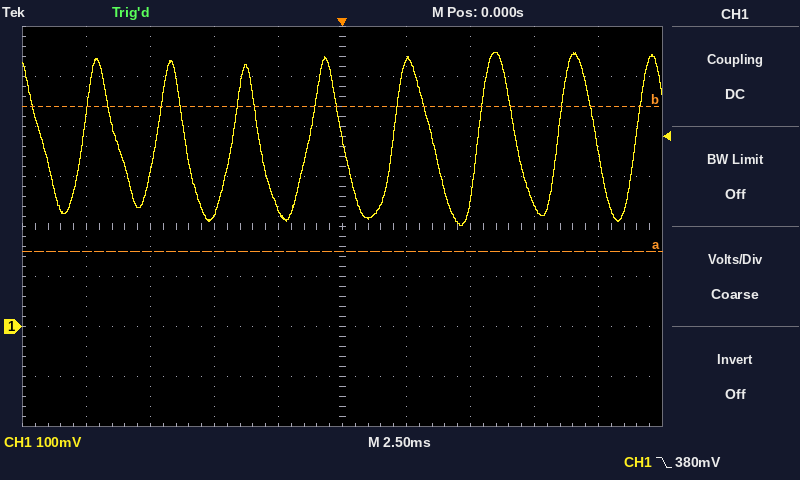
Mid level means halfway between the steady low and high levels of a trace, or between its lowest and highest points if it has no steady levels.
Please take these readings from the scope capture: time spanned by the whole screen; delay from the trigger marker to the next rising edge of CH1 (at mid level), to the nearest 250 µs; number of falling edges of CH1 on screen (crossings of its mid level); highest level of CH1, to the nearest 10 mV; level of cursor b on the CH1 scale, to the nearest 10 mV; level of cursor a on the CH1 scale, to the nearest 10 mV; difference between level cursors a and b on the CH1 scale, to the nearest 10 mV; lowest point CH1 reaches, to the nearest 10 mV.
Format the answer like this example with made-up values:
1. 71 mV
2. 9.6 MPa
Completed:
1. 25 ms
2. 2.00 ms
3. 8
4. 550 mV
5. 440 mV
6. 150 mV
7. 290 mV
8. 200 mV
